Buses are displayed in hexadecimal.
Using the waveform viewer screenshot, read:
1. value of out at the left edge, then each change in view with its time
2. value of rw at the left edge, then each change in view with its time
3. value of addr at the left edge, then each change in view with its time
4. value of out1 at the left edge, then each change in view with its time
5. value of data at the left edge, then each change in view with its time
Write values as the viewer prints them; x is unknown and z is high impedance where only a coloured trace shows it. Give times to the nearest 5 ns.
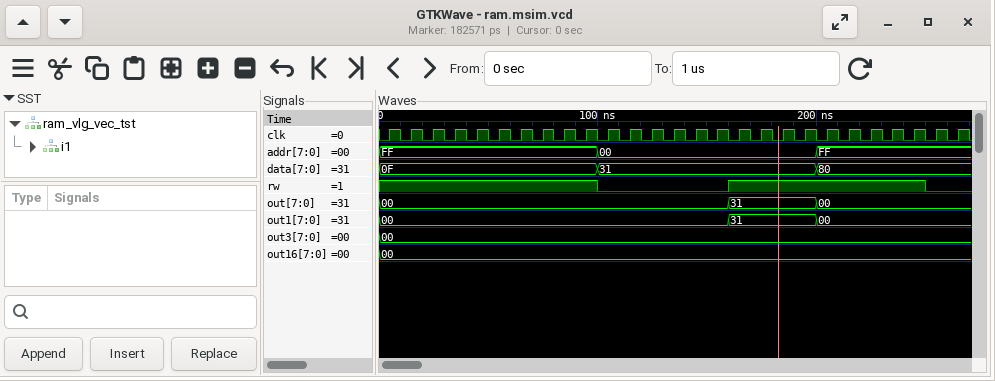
00, 31 at 160 ns, 00 at 200 ns
1, 0 at 100 ns, 1 at 160 ns, 0 at 250 ns
FF, 00 at 100 ns, FF at 200 ns
00, 31 at 160 ns, 00 at 200 ns
0F, 31 at 100 ns, 80 at 200 ns
